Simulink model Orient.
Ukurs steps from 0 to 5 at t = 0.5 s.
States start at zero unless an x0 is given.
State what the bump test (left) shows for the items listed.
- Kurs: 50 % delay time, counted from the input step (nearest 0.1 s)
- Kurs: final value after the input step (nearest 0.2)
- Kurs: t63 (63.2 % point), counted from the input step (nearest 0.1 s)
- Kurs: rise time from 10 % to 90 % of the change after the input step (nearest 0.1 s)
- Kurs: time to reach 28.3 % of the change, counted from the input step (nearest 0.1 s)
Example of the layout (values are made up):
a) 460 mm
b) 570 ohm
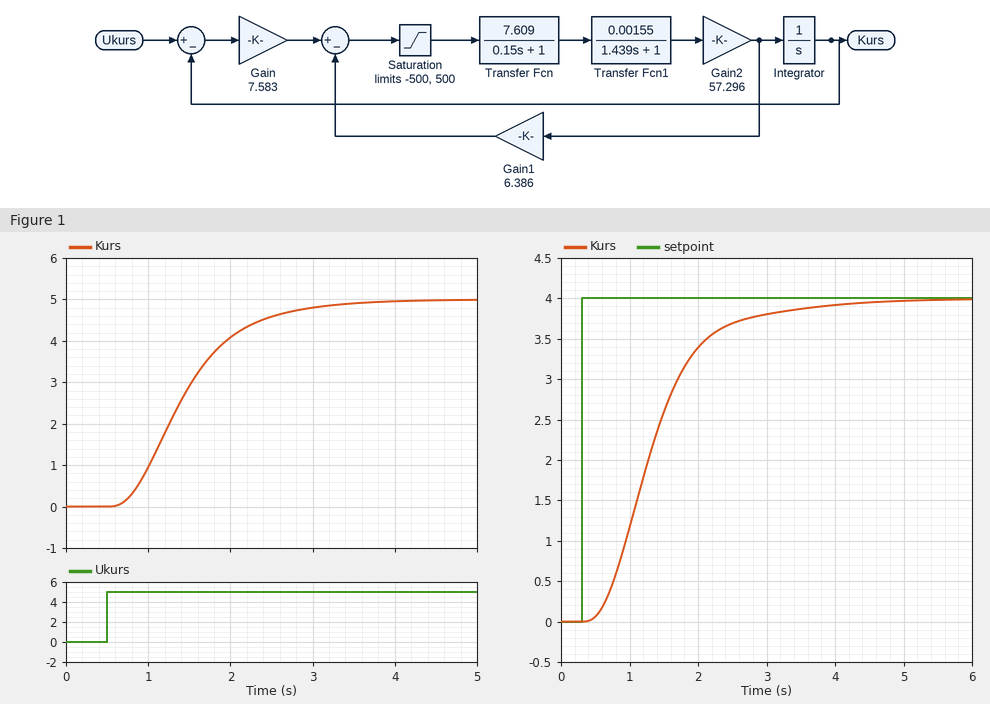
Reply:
a) 0.9 s
b) 5.0
c) 1.1 s
d) 1.5 s
e) 0.6 s
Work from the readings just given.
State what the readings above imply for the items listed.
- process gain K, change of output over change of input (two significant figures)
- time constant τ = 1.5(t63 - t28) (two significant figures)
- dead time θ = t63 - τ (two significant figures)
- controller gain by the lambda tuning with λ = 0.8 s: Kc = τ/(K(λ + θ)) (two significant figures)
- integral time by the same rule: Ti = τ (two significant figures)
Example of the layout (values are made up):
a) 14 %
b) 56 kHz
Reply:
a) 1.0
b) 0.75 s
c) 0.35 s
d) 0.65
e) 0.75 s
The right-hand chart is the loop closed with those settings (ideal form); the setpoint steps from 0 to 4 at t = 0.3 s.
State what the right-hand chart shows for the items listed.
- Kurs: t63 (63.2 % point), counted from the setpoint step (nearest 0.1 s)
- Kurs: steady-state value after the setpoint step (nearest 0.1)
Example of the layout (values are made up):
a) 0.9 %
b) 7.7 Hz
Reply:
a) 1.2 s
b) 4.0
